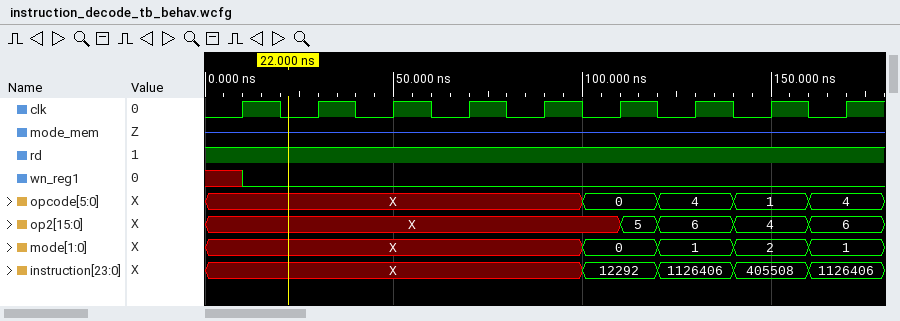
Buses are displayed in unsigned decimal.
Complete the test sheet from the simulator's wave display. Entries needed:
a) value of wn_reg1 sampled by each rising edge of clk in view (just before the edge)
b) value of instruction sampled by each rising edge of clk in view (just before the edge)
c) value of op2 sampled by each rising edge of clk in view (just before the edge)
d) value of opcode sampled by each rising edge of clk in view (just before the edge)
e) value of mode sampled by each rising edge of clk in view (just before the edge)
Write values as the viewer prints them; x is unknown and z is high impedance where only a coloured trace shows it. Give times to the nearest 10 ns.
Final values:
x 0 0 0 0 0 0 0 0
X, X, X, X, X, 12292, 1126406, 405508, 1126406
X, X, X, X, X, X, 6, 4, 6
X, X, X, X, X, 0, 4, 1, 4
X, X, X, X, X, 0, 1, 2, 1
